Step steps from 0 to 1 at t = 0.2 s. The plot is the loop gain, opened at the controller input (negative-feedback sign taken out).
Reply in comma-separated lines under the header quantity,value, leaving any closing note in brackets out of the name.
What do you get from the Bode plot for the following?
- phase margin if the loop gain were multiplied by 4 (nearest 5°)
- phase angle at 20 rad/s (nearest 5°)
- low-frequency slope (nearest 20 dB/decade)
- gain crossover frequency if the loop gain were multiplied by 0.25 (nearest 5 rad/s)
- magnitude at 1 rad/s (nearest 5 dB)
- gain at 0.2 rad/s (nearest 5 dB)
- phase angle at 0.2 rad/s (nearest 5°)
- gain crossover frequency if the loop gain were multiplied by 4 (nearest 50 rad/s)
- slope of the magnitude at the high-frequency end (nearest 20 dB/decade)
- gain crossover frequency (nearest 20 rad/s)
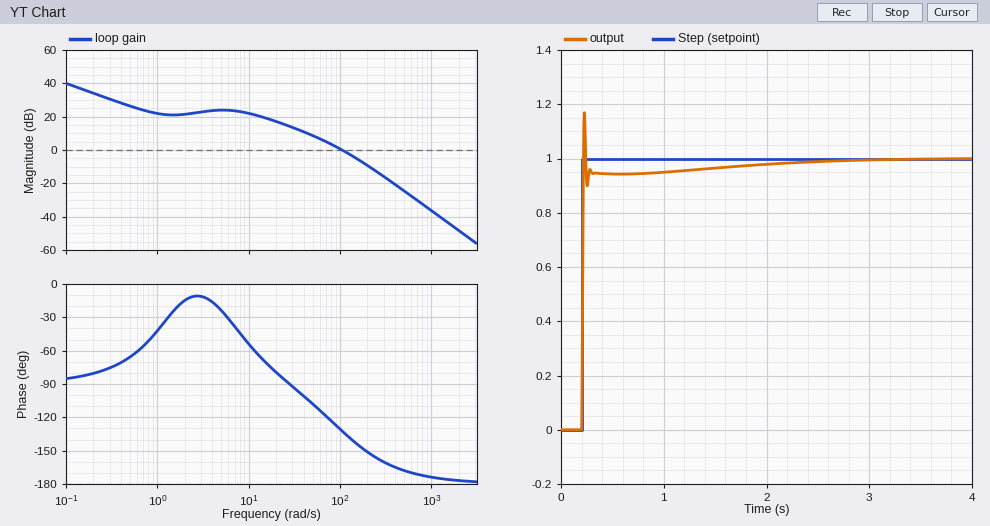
quantity,value
phase margin if the loop gain were multiplied by 4,25°
phase angle at 20 rad/s,-80°
low-frequency slope,-20 dB/decade
gain crossover frequency if the loop gain were multiplied by 0.25,35 rad/s
magnitude at 1 rad/s,20 dB
gain at 0.2 rad/s,35 dB
phase angle at 0.2 rad/s,-80°
gain crossover frequency if the loop gain were multiplied by 4,250 rad/s
slope of the magnitude at the high-frequency end,-40 dB/decade
gain crossover frequency,100 rad/s
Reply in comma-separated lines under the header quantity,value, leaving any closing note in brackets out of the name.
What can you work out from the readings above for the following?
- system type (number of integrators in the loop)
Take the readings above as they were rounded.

quantity,value
system type,1
